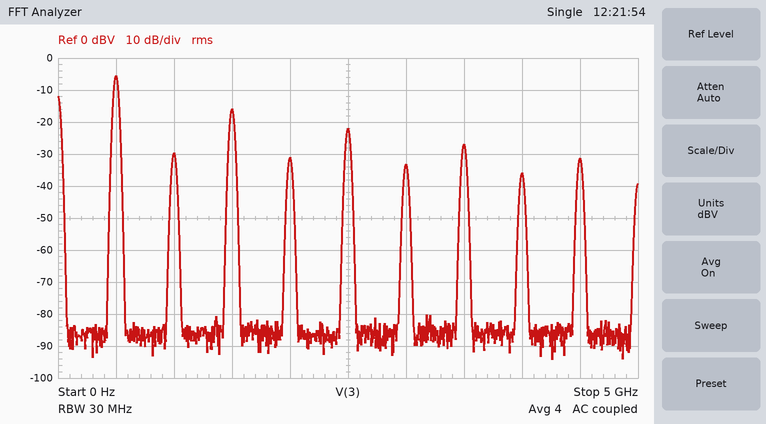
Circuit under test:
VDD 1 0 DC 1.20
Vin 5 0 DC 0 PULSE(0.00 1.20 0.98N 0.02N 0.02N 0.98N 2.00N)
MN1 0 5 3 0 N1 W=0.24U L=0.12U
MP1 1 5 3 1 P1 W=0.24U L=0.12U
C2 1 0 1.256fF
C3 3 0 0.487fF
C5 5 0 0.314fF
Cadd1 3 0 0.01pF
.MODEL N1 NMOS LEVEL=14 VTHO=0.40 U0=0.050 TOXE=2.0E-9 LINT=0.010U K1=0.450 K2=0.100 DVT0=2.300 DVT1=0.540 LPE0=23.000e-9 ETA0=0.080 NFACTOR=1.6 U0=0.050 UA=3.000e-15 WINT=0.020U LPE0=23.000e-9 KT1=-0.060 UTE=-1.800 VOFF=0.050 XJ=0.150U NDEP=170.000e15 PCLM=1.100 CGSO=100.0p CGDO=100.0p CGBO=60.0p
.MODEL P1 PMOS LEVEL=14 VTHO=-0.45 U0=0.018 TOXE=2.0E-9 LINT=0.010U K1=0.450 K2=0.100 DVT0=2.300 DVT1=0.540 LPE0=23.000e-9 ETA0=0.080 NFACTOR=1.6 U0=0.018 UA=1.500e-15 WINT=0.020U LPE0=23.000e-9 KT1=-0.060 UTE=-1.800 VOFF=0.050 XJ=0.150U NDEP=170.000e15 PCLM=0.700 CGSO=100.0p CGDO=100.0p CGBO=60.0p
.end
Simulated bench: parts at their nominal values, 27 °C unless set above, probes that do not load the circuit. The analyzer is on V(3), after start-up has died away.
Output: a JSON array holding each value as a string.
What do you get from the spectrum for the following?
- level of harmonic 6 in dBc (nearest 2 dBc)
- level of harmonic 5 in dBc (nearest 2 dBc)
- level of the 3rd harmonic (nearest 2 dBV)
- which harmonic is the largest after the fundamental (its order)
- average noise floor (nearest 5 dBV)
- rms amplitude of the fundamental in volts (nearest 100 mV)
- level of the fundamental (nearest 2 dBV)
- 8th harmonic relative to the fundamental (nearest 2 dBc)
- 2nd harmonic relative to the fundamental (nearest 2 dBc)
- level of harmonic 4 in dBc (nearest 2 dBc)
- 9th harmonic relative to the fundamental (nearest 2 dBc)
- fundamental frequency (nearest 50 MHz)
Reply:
["-28 dBc", "-16 dBc", "-16 dBV", "3", "-85 dBV", "500 mV", "-6 dBV", "-30 dBc", "-24 dBc", "-26 dBc", "-26 dBc", "500 MHz"]
